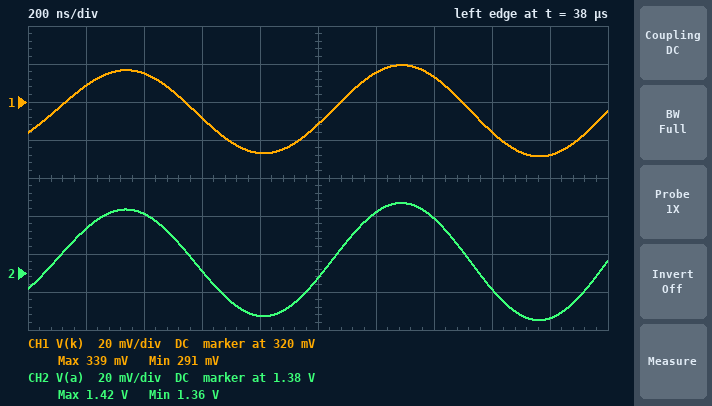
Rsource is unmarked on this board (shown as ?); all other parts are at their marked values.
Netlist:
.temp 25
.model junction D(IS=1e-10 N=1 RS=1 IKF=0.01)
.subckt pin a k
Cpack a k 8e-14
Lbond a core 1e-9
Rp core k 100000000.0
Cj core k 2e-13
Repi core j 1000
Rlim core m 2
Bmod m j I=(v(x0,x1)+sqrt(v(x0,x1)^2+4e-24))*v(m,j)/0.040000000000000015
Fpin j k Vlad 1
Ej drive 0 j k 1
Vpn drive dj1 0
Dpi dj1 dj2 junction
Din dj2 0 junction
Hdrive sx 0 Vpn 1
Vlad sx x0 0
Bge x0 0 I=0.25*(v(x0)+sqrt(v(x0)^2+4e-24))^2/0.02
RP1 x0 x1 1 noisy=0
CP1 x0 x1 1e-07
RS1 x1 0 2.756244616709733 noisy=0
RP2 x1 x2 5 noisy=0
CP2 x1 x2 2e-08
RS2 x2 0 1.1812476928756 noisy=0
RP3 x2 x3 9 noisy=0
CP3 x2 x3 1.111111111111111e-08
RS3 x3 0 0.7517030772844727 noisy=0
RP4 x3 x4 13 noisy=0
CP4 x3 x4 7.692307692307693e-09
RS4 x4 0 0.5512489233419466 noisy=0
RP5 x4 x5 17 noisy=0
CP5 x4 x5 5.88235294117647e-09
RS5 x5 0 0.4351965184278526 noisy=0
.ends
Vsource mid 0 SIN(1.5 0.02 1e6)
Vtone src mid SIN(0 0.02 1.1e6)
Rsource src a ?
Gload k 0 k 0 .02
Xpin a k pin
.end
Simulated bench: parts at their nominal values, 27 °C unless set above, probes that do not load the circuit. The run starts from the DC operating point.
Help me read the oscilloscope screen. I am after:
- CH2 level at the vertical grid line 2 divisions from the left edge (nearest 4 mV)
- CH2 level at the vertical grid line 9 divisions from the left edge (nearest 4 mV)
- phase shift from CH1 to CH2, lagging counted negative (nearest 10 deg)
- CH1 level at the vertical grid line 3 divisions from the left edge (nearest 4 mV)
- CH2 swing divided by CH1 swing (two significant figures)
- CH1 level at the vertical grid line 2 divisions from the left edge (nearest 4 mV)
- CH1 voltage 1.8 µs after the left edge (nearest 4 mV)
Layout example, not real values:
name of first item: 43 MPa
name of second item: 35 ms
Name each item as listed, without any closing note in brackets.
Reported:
CH2 level at the vertical grid line 2 divisions from the left edge: 1.412 V
CH2 level at the vertical grid line 9 divisions from the left edge: 1.356 V
phase shift from CH1 to CH2, lagging counted negative: 0 deg
CH1 level at the vertical grid line 3 divisions from the left edge: 312 mV
CH2 swing divided by CH1 swing: 1.3
CH1 level at the vertical grid line 2 divisions from the left edge: 336 mV
CH1 voltage 1.8 µs after the left edge: 292 mV
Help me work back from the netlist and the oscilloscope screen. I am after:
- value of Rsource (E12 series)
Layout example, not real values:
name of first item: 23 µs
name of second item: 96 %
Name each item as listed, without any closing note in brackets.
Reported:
value of Rsource: 18 Ω
